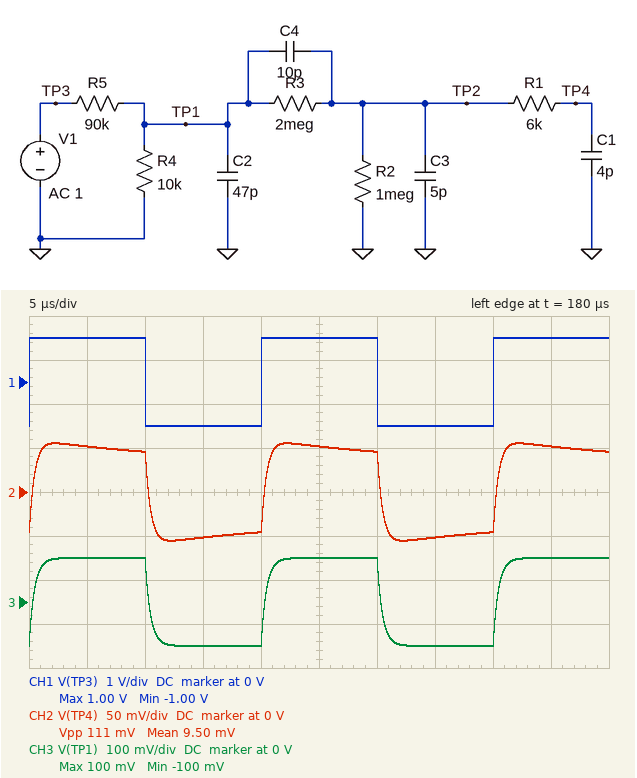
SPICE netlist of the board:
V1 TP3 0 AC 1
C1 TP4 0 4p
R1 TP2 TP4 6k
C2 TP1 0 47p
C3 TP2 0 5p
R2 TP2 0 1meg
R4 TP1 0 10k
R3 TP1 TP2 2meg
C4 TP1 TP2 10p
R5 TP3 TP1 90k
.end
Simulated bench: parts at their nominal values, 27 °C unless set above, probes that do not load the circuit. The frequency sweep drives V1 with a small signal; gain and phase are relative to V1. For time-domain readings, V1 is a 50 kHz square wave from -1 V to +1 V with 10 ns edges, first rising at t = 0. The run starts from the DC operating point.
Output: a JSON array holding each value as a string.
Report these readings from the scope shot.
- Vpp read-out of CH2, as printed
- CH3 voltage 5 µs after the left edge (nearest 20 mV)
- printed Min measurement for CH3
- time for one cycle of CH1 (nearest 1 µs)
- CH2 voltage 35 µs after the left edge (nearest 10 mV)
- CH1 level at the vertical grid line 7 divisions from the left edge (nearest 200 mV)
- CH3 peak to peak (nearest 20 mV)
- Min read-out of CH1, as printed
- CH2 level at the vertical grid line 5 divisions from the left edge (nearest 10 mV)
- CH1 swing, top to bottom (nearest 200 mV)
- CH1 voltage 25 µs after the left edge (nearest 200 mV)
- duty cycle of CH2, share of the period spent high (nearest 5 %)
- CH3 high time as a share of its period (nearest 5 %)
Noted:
["111 mV", "100 mV", "-100 mV", "20 µs", "-50 mV", "-1.0 V", "200 mV", "-1.00 V", "50 mV", "2.0 V", "1.0 V", "50 %", "50 %"]
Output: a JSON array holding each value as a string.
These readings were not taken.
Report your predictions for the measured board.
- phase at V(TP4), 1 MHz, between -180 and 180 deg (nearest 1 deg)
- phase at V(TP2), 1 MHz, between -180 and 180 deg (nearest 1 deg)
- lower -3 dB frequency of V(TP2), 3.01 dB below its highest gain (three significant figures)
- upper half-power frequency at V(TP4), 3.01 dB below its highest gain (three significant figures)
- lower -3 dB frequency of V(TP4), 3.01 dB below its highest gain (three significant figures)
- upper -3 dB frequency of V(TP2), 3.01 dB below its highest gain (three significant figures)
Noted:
["-77 deg", "-69 deg", "4.62 kHz", "361 kHz", "4.62 kHz", "362 kHz"]
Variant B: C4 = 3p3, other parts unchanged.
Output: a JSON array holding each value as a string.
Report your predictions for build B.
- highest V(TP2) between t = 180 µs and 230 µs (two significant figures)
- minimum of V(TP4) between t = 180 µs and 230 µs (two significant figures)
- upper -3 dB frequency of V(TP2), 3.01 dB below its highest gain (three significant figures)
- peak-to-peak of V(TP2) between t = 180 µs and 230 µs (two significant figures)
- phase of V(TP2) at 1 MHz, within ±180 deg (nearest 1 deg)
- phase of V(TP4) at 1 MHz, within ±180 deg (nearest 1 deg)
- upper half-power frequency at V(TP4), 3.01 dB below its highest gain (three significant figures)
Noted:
["30 mV", "-30 mV", "197 kHz", "60 mV", "-68 deg", "-76 deg", "196 kHz"]
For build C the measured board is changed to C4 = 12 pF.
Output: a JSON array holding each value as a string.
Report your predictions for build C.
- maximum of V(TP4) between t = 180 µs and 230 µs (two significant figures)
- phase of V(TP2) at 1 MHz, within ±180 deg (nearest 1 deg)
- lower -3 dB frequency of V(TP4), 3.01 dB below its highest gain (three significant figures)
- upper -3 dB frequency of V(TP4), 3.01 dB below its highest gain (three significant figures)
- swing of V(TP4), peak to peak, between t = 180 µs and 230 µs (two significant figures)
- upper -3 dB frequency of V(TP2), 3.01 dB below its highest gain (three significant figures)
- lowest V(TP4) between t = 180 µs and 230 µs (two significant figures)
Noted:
["60 mV", "-69 deg", "5.72 kHz", "357 kHz", "120 mV", "358 kHz", "-60 mV"]
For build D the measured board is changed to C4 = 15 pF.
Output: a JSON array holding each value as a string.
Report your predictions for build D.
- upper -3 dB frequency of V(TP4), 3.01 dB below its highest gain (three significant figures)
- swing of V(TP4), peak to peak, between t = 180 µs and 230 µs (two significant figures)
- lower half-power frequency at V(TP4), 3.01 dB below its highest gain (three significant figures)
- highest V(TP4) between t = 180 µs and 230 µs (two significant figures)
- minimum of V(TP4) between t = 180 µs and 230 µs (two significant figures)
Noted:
["353 kHz", "130 mV", "6.00 kHz", "66 mV", "-66 mV"]
